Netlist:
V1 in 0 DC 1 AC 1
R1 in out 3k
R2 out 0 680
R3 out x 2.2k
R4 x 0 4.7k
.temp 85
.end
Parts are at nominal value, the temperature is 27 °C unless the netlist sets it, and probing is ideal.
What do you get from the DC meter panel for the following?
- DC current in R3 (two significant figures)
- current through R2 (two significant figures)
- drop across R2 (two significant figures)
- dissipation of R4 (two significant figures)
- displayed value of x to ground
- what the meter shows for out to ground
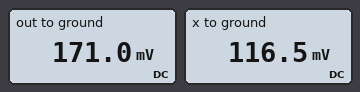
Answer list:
25 µA
250 µA
170 mV
2.9 µW
116.5 mV
171.0 mV
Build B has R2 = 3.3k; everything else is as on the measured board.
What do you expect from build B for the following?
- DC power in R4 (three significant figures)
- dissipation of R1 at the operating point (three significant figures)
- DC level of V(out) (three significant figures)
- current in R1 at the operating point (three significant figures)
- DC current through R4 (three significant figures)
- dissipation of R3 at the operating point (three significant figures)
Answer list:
18.0 µW
110 µW
427 mV
191 µA
61.8 µA
8.41 µW
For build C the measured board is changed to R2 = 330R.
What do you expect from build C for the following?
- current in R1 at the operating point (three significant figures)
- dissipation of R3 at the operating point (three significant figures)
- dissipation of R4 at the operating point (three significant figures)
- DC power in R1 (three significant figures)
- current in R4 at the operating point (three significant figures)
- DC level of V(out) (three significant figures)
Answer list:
302 µA
417 nW
891 nW
273 µW
13.8 µA
95.0 mV
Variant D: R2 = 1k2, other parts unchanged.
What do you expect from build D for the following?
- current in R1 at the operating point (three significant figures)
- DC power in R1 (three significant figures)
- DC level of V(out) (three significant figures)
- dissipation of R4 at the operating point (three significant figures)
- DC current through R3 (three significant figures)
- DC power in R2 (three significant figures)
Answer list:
249 µA
185 µW
254 mV
6.38 µW
36.8 µA
53.8 µW
